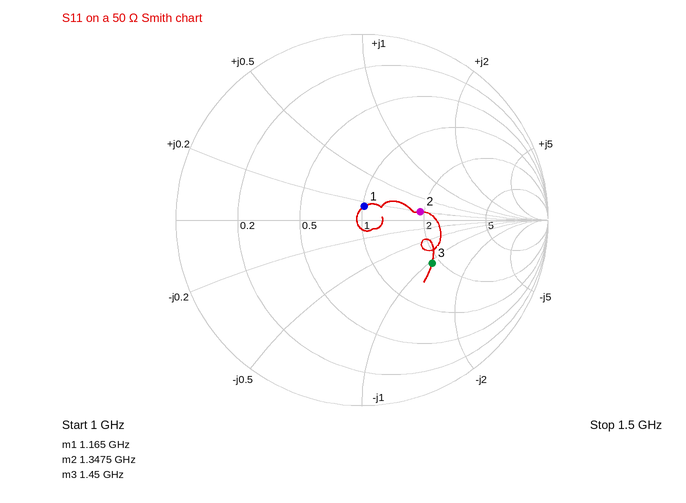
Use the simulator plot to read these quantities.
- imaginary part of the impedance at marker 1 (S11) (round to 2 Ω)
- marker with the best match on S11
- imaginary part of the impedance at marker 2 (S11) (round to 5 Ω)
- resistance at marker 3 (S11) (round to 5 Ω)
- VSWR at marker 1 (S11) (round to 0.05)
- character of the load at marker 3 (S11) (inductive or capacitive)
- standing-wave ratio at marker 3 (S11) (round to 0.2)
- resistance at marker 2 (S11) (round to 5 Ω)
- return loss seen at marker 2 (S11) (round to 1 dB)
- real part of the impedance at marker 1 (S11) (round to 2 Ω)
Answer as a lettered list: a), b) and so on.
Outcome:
a) +8 Ω
b) marker 1
c) +10 Ω
d) 90 Ω
e) 1.15
f) capacitive
g) 2.6
h) 95 Ω
i) 10 dB
j) 50 Ω
